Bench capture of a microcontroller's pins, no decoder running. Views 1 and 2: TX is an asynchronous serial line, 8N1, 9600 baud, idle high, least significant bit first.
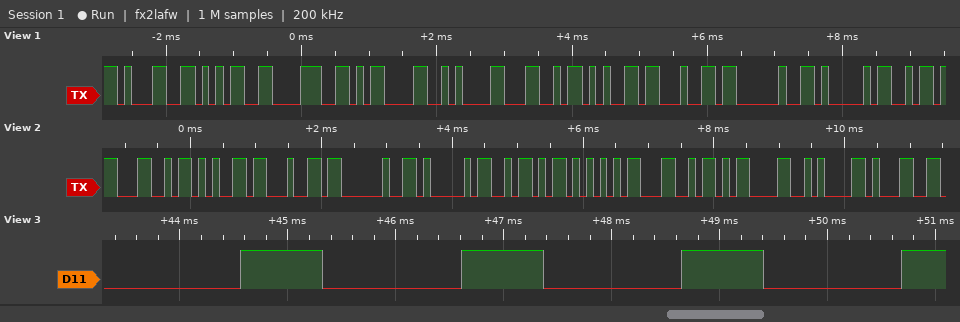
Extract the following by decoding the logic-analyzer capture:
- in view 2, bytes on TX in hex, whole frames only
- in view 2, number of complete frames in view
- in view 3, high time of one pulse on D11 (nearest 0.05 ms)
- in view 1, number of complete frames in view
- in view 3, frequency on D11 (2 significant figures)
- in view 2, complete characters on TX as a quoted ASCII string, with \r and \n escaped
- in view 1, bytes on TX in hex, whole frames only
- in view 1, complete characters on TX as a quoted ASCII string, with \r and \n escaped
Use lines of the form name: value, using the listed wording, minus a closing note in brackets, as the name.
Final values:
in view 2, bytes on TX in hex, whole frames only: 4C 65 64 20 41 5A 55 4C 0D 0A 31
in view 2, number of complete frames in view: 11
in view 3, high time of one pulse on D11: 0.75 ms
in view 1, number of complete frames in view: 10
in view 3, frequency on D11: 490 Hz
in view 2, complete characters on TX as a quoted ASCII string, with \r and \n escaped: "Led AZUL\r\n1"
in view 1, bytes on TX in hex, whole frames only: 0x31 0x35 0x38 0x0D 0x0A 0x4C 0x65 0x64 0x20 0x41
in view 1, complete characters on TX as a quoted ASCII string, with \r and \n escaped: "158\r\nLed A"
